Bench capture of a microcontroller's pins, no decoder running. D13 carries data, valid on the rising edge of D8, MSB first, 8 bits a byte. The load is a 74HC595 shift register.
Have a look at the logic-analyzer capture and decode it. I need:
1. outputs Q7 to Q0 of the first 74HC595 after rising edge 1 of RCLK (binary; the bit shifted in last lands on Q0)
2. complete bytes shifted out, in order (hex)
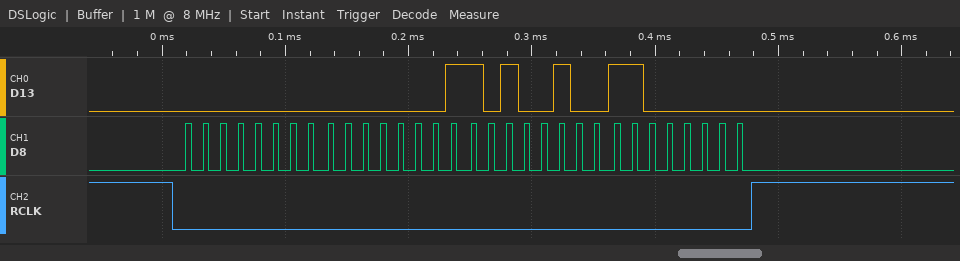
11000000
00 01 A4 C0
